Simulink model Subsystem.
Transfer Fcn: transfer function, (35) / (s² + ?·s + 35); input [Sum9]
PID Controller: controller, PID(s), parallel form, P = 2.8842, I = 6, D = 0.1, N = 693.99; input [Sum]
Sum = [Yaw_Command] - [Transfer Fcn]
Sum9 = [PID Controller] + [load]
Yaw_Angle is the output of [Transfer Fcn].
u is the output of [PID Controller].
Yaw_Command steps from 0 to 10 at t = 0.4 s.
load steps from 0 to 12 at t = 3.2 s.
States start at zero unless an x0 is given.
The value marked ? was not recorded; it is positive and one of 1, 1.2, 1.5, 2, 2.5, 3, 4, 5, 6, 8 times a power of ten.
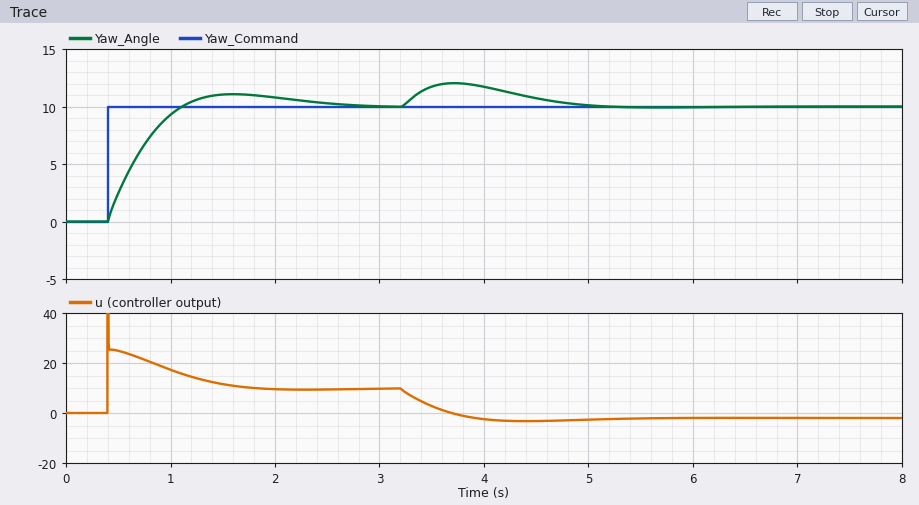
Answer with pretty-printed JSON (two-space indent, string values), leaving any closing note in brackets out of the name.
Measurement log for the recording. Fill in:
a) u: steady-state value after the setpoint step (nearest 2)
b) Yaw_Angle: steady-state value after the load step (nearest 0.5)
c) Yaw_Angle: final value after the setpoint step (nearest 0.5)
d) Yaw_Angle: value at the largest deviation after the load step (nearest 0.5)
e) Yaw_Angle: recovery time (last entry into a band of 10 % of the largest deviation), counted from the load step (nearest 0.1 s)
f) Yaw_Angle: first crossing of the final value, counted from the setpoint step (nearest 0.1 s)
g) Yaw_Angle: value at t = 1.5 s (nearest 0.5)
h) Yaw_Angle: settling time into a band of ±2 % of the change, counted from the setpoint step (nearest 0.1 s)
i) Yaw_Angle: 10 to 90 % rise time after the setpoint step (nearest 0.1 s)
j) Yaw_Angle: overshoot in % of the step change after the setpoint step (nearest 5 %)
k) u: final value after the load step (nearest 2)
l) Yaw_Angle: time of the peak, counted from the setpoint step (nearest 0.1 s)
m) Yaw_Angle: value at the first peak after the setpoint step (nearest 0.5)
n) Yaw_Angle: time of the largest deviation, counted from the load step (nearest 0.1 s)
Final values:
{
  "u: steady-state value after the setpoint step": "10",
  "Yaw_Angle: steady-state value after the load step": "10.0",
  "Yaw_Angle: final value after the setpoint step": "10.0",
  "Yaw_Angle: value at the largest deviation after the load step": "12.0",
  "Yaw_Angle: recovery time (last entry into a band of 10 % of the largest deviation), counted from the load step": "1.7 s",
  "Yaw_Angle: first crossing of the final value, counted from the setpoint step": "0.7 s",
  "Yaw_Angle: value at t = 1.5 s": "11.0",
  "Yaw_Angle: settling time into a band of ±2 % of the change, counted from the setpoint step": "2.2 s",
  "Yaw_Angle: 10 to 90 % rise time after the setpoint step": "0.5 s",
  "Yaw_Angle: overshoot in % of the step change after the setpoint step": "10 %",
  "u: final value after the load step": "-2",
  "Yaw_Angle: time of the peak, counted from the setpoint step": "1.2 s",
  "Yaw_Angle: value at the first peak after the setpoint step": "11.0",
  "Yaw_Angle: time of the largest deviation, counted from the load step": "0.5 s"
}
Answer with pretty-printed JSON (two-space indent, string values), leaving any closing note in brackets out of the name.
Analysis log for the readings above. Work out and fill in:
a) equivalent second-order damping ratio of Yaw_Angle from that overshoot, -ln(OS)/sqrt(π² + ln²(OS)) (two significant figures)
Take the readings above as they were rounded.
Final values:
{
  "equivalent second-order damping ratio of Yaw_Angle from that overshoot, -ln(OS)/sqrt(π² + ln²(OS))": "0.59"
}
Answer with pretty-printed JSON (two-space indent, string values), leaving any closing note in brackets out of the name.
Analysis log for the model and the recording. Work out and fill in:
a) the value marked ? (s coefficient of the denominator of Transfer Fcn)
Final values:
{
  "the value marked ?": "40"
}
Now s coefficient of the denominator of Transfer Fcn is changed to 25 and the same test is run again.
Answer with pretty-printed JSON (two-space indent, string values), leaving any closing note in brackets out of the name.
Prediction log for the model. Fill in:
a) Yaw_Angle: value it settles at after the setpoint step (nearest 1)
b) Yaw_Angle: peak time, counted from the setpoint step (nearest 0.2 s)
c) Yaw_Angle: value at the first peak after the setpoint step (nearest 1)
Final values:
{
  "Yaw_Angle: value it settles at after the setpoint step": "10",
  "Yaw_Angle: peak time, counted from the setpoint step": "1.0 s",
  "Yaw_Angle: value at the first peak after the setpoint step": "10"
}
